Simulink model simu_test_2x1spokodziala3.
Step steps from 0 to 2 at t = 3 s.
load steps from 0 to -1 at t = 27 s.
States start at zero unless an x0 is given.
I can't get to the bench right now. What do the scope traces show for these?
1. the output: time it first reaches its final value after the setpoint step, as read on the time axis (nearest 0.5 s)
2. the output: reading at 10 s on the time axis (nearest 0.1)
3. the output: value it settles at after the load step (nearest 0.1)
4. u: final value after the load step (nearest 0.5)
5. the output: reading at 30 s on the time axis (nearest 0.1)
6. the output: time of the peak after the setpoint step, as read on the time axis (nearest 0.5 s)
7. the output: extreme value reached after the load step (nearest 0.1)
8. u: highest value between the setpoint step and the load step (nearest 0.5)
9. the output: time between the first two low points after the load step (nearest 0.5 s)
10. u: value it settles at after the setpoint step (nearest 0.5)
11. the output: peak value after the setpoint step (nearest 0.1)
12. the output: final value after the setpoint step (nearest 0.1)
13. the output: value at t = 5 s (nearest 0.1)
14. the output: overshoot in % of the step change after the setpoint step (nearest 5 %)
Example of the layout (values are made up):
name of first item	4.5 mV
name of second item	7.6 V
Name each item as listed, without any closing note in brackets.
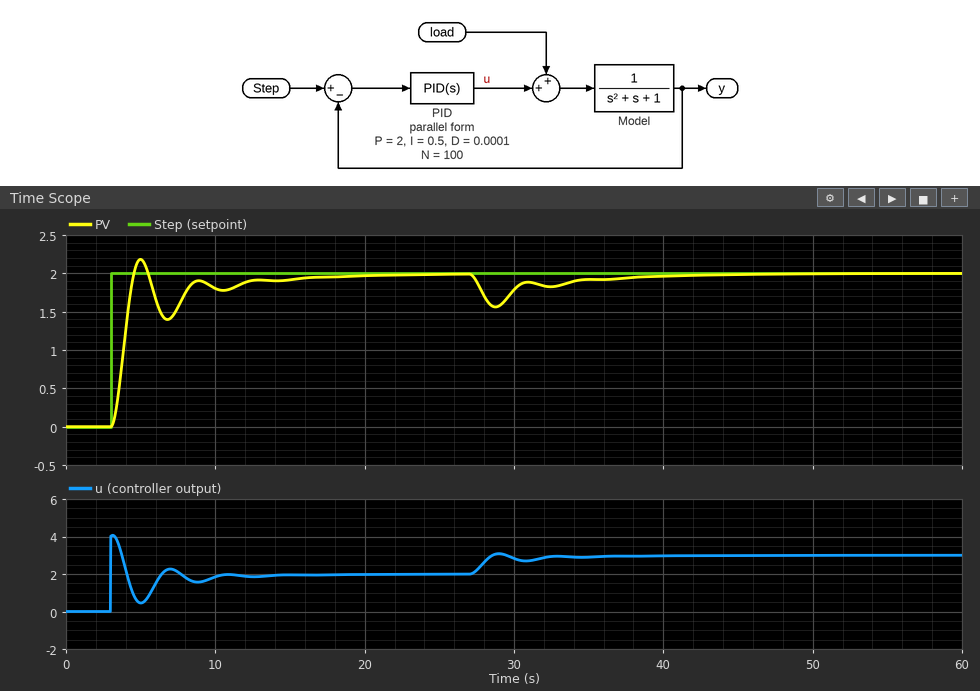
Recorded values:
the output: time it first reaches its final value after the setpoint step, as read on the time axis	4.5 s
the output: reading at 10 s on the time axis	1.8
the output: value it settles at after the load step	2.0
u: final value after the load step	3.0
the output: reading at 30 s on the time axis	1.8
the output: time of the peak after the setpoint step, as read on the time axis	5.0 s
the output: extreme value reached after the load step	1.6
u: highest value between the setpoint step and the load step	4.0
the output: time between the first two low points after the load step	3.5 s
u: value it settles at after the setpoint step	2.0
the output: peak value after the setpoint step	2.2
the output: final value after the setpoint step	2.0
the output: value at t = 5 s	2.2
the output: overshoot in % of the step change after the setpoint step	10 %
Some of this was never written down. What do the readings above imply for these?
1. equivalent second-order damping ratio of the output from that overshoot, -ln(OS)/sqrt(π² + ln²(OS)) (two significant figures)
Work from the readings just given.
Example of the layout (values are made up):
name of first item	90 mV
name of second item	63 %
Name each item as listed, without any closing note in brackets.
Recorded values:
equivalent second-order damping ratio of the output from that overshoot, -ln(OS)/sqrt(π² + ln²(OS))	0.59
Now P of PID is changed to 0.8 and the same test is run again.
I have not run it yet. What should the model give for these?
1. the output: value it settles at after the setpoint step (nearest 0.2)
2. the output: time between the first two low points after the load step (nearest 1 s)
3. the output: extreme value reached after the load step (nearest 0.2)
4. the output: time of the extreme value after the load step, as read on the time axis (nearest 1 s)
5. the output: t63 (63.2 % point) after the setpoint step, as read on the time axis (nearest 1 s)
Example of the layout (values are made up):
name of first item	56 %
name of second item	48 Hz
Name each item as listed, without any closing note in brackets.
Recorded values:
the output: value it settles at after the setpoint step	2.0
the output: time between the first two low points after the load step	5 s
the output: extreme value reached after the load step	1.4
the output: time of the extreme value after the load step, as read on the time axis	29 s
the output: t63 (63.2 % point) after the setpoint step, as read on the time axis	5 s
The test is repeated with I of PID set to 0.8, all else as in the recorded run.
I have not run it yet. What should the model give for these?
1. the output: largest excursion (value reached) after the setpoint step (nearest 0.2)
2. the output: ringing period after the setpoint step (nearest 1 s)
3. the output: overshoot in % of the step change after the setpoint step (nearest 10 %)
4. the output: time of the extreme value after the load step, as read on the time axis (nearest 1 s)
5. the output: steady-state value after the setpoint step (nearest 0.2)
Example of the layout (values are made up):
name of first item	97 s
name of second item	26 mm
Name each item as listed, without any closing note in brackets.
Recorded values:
the output: largest excursion (value reached) after the setpoint step	2.4
the output: ringing period after the setpoint step	4 s
the output: overshoot in % of the step change after the setpoint step	20 %
the output: time of the extreme value after the load step, as read on the time axis	29 s
the output: steady-state value after the setpoint step	2.0
